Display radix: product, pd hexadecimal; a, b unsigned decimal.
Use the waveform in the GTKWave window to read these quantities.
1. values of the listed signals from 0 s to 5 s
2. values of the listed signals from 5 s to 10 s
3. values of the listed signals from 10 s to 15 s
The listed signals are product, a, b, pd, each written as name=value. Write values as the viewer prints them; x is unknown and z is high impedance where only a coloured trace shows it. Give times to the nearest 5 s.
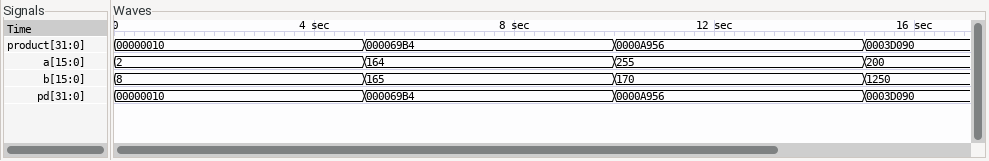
product=00000010, a=2, b=8, pd=00000010
product=000069B4, a=164, b=165, pd=000069B4
product=0000A956, a=255, b=170, pd=0000A956
